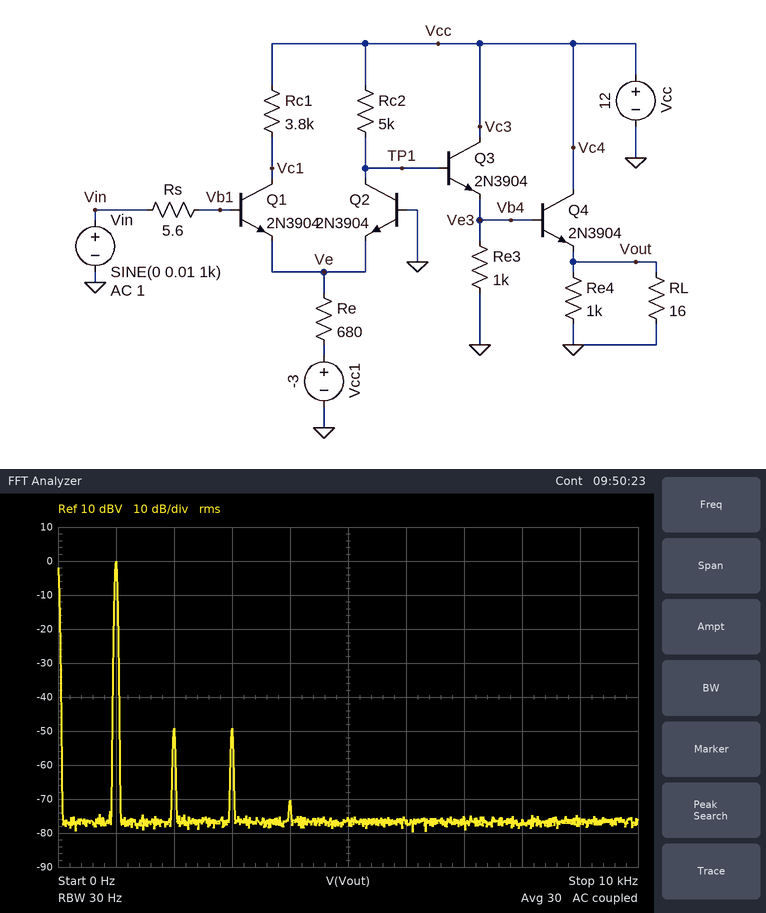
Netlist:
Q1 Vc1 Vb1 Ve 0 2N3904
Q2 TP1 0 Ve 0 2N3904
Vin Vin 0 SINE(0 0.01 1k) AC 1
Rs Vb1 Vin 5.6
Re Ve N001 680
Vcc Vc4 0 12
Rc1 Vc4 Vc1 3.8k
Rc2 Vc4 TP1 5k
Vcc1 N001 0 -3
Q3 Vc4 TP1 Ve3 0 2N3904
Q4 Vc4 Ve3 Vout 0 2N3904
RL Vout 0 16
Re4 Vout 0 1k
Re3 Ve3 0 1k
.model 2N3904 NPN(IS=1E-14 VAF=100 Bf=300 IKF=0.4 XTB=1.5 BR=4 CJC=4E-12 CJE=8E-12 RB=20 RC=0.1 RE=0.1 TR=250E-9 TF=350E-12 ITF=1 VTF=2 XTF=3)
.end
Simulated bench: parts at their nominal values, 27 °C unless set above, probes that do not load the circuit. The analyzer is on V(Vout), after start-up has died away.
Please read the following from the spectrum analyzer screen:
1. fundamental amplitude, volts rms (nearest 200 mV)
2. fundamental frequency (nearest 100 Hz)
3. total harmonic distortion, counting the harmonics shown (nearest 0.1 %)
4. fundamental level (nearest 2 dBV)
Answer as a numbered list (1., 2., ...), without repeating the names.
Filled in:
1. 1.0 V
2. 1.0 kHz
3. 0.5 %
4. 0 dBV
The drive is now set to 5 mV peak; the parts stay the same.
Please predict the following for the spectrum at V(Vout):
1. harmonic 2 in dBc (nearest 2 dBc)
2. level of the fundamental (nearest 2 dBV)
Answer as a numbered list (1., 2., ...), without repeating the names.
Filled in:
1. -58 dBc
2. -6 dBV
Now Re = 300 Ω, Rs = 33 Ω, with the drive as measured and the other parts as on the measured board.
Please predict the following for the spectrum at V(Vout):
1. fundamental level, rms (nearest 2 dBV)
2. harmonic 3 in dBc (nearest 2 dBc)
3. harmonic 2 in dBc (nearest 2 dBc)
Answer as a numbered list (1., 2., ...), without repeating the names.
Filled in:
1. -180 dBV
2. 0 dBc
3. 0 dBc
